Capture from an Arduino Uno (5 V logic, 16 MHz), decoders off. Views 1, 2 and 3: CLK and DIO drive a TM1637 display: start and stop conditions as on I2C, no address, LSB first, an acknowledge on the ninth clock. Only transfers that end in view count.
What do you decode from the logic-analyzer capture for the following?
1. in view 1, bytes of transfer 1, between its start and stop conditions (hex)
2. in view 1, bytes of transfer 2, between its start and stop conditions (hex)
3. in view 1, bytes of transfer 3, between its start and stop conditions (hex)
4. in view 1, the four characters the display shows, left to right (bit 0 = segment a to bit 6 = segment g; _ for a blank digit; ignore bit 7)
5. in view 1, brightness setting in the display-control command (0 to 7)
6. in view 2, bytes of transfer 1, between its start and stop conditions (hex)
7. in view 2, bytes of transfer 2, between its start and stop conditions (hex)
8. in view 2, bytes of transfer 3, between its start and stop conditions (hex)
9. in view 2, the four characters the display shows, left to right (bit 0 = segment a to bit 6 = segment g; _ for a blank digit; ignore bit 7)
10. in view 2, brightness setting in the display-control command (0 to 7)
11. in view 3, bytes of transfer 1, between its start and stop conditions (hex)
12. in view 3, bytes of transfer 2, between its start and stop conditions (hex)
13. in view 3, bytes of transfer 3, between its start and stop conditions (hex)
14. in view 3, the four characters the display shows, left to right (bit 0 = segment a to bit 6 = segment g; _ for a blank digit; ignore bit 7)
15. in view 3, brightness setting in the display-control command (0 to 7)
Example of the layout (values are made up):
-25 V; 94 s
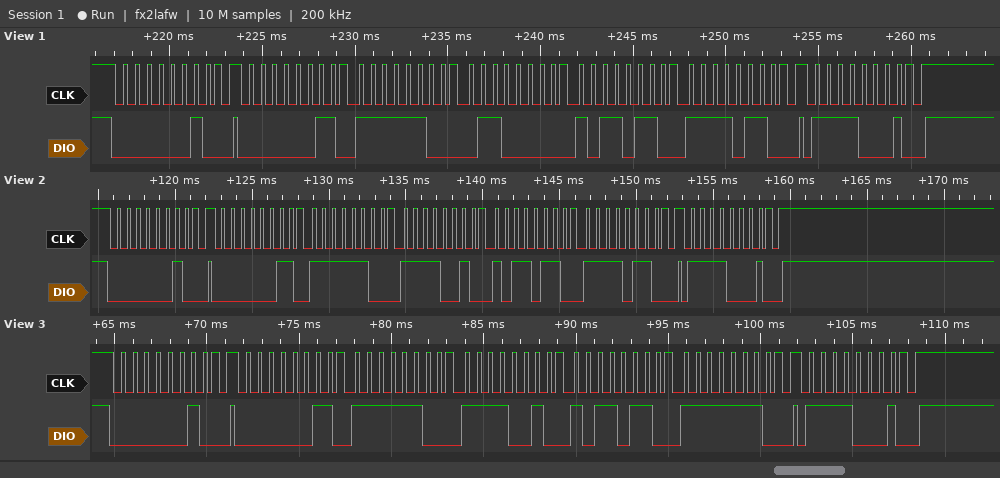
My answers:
40; C0 3F 06 6D 6F; 8F; 0159; 7; 40; C0 3F 4F 6D 6F; 8F; 0359; 7; 40; C0 3F 4F 6D 7F; 8F; 0358; 7
